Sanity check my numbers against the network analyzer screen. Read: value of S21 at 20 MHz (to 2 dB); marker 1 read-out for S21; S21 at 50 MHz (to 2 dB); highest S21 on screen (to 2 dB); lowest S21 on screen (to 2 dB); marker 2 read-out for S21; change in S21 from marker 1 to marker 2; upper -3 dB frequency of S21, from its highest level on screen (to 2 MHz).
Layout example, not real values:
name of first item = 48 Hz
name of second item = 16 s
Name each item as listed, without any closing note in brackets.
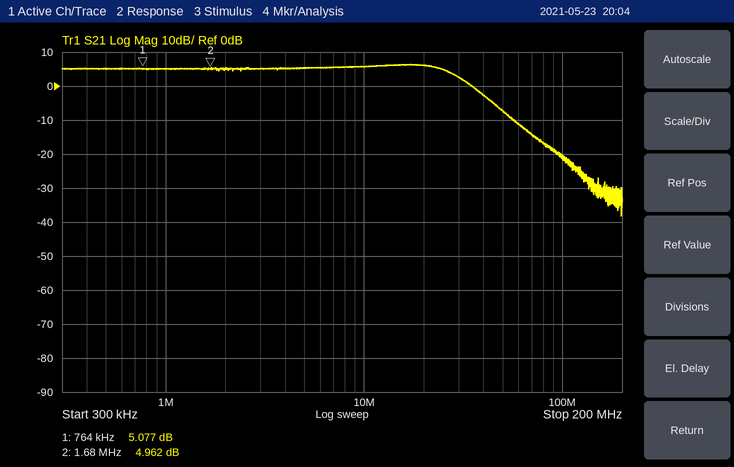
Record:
value of S21 at 20 MHz = 6 dB
marker 1 read-out for S21 = 5.077 dB
S21 at 50 MHz = -8 dB
highest S21 on screen = 6 dB
lowest S21 on screen = -38 dB
marker 2 read-out for S21 = 4.962 dB
change in S21 from marker 1 to marker 2 = -0.115 dB
upper -3 dB frequency of S21, from its highest level on screen = 28 MHz
